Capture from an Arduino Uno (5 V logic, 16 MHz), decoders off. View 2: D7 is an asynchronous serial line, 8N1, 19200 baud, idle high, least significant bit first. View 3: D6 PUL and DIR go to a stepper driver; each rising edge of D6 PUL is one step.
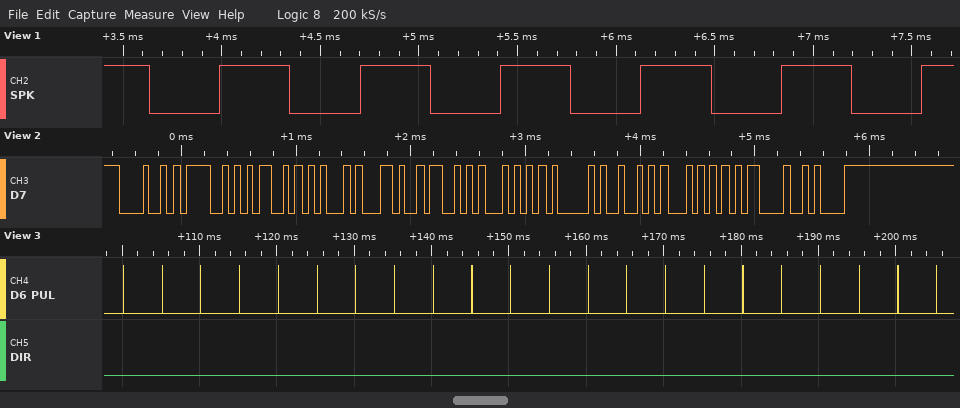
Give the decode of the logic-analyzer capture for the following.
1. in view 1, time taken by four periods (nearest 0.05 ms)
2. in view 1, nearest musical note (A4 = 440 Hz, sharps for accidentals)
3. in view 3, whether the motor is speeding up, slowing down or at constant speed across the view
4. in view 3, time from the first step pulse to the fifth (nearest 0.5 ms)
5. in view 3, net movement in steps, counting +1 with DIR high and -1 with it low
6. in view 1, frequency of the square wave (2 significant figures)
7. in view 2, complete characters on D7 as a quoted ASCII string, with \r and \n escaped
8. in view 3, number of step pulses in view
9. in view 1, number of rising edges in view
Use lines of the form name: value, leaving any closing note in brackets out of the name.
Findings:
in view 1, time taken by four periods: 2.85 ms
in view 1, nearest musical note: F6
in view 3, whether the motor is speeding up, slowing down or at constant speed across the view: constant speed
in view 3, time from the first step pulse to the fifth: 20.0 ms
in view 3, net movement in steps, counting +1 with DIR high and -1 with it low: -22
in view 1, frequency of the square wave: 1.4 kHz
in view 2, complete characters on D7 as a quoted ASCII string, with \r and \n escaped: "HOME,START\r\n"
in view 3, number of step pulses in view: 22
in view 1, number of rising edges in view: 6
